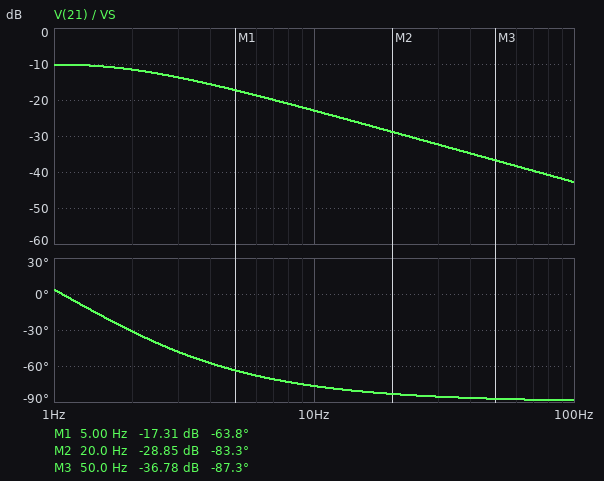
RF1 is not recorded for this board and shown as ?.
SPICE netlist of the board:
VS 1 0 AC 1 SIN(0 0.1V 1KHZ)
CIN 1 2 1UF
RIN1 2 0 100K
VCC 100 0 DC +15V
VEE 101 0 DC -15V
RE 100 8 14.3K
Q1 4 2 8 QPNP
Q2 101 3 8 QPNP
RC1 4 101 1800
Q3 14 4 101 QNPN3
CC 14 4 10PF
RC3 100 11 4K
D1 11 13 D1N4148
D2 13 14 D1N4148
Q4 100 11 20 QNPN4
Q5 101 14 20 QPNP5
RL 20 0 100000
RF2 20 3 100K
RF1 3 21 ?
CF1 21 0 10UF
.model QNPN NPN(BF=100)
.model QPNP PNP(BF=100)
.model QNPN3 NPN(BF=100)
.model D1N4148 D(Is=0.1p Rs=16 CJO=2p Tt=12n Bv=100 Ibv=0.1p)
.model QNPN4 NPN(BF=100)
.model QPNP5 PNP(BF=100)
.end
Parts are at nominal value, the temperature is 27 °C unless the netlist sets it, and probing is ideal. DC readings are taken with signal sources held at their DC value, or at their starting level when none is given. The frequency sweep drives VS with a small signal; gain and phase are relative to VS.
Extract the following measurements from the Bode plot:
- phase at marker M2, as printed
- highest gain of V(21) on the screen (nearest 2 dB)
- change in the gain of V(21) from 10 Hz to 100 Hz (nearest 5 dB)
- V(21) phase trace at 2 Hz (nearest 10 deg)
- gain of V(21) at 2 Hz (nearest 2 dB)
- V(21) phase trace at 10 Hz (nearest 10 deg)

-83.3 deg
-10 dB
-20 dB
-30 deg
-12 dB
-80 deg
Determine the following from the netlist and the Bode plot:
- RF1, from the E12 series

22 kΩ
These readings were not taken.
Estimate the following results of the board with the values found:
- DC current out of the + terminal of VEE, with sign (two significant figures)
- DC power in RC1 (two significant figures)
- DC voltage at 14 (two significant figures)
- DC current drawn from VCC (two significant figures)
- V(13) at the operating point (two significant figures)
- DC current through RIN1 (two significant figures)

-4.6 mA
360 µW
-670 mV
4.6 mA
15 mV
4.8 µA
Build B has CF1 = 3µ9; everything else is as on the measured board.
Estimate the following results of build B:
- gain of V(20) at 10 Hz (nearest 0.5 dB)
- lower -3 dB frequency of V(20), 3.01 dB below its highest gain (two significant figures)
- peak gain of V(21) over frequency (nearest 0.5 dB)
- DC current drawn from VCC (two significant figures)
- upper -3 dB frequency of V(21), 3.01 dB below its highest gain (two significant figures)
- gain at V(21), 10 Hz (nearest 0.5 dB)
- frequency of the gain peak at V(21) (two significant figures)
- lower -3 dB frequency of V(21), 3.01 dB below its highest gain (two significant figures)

14.5 dB
2.7 Hz
-5.5 dB
4.6 mA
4.2 Hz
-15.0 dB
1.7 Hz
710 mHz
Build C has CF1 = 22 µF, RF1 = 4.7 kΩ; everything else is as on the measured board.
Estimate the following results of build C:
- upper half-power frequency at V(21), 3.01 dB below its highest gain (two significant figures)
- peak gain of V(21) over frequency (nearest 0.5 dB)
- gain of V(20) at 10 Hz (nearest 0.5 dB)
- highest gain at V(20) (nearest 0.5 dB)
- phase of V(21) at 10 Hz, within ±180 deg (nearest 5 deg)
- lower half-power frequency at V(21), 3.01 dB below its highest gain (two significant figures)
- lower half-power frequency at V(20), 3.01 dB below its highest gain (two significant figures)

3.9 Hz
-6.5 dB
26.5 dB
27.0 dB
-70 deg
630 mHz
2.6 Hz
